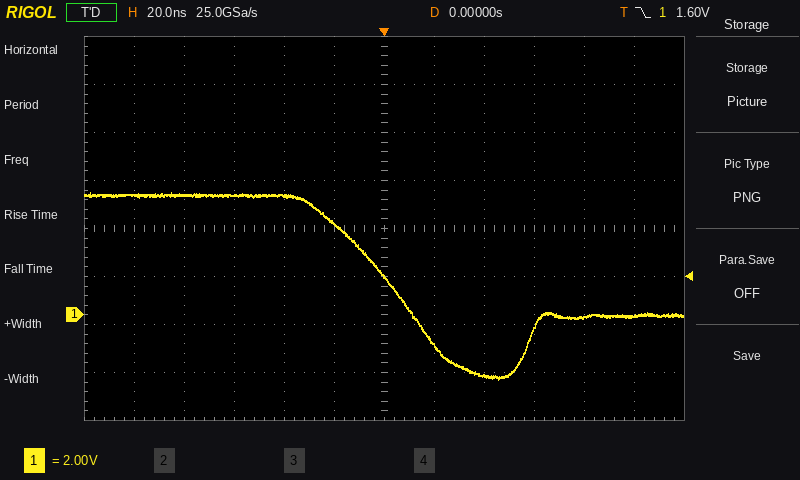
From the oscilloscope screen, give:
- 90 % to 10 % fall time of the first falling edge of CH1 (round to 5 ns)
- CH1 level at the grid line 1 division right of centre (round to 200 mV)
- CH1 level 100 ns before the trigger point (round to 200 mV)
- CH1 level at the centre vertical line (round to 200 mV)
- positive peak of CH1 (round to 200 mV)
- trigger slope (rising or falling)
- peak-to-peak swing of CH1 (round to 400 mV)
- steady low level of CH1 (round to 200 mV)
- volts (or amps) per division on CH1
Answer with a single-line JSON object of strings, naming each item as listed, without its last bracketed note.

{"90 % to 10 % fall time of the first falling edge of CH1": "35 ns", "CH1 level at the grid line 1 division right of centre": "-1.2 V", "CH1 level 100 ns before the trigger point": "5.0 V", "CH1 level at the centre vertical line": "1.6 V", "positive peak of CH1": "5.0 V", "trigger slope": "falling", "peak-to-peak swing of CH1": "7.6 V", "steady low level of CH1": "0.0 V", "volts (or amps) per division on CH1": "2 V"}
